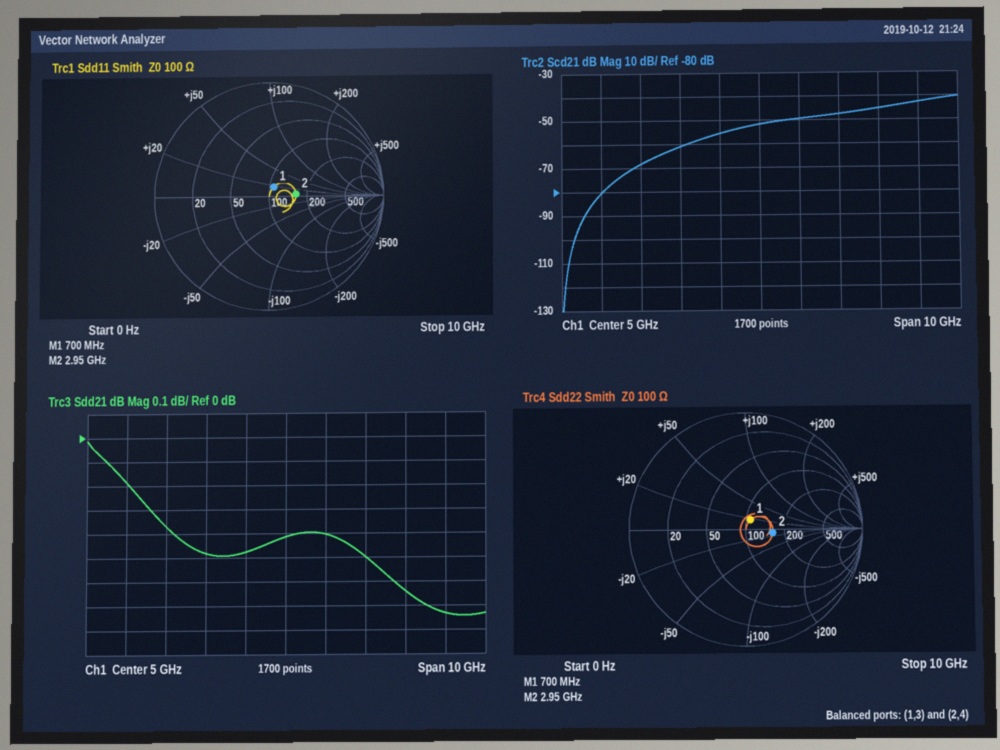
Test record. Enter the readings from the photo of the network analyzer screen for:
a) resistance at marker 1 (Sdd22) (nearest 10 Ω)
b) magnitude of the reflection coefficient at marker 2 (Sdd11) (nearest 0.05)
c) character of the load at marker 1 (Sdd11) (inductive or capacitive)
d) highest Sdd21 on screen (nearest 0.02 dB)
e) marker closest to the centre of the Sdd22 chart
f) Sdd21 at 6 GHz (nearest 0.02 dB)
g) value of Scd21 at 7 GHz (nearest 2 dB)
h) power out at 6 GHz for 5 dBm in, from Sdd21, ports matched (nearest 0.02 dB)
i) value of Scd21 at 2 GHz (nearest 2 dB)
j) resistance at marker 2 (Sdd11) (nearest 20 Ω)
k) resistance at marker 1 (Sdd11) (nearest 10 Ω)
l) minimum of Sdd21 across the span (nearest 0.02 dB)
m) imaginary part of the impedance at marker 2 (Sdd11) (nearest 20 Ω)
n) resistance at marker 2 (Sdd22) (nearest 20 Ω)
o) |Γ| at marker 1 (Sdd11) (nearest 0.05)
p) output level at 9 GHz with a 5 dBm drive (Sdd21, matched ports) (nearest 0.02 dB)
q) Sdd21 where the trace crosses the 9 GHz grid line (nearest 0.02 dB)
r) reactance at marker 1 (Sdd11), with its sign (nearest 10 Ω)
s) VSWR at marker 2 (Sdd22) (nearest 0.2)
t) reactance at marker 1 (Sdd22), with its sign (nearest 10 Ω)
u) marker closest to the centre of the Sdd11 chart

110 Ω
0.25
inductive
-0.02 dB
marker 1
-0.40 dB
-48 dB
4.60 dBm
-68 dB
160 Ω
110 Ω
-0.74 dB
0 Ω
160 Ω
0.10
4.26 dBm
-0.74 dB
+20 Ω
1.6
+20 Ω
marker 1
